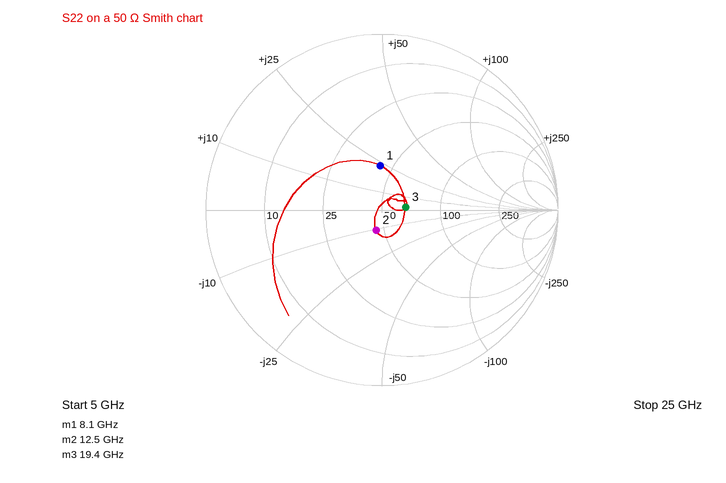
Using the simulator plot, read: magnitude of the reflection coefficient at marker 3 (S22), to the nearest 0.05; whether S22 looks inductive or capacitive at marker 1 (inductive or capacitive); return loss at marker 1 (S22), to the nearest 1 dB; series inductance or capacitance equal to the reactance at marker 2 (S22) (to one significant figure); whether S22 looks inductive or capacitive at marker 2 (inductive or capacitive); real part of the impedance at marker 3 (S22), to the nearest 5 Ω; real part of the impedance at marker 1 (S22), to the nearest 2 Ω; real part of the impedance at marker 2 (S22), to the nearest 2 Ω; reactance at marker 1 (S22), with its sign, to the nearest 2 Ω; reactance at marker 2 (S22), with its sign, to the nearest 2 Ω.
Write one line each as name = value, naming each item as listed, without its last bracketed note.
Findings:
magnitude of the reflection coefficient at marker 3 (S22), to the nearest 0.05 = 0.15
whether S22 looks inductive or capacitive at marker 1 = inductive
return loss at marker 1 (S22), to the nearest 1 dB = 12 dB
series inductance or capacitance equal to the reactance at marker 2 (S22) = 1 pF
whether S22 looks inductive or capacitive at marker 2 = capacitive
real part of the impedance at marker 3 (S22), to the nearest 5 Ω = 65 Ω
real part of the impedance at marker 1 (S22), to the nearest 2 Ω = 44 Ω
real part of the impedance at marker 2 (S22), to the nearest 2 Ω = 46 Ω
reactance at marker 1 (S22), with its sign, to the nearest 2 Ω = +24 Ω
reactance at marker 2 (S22), with its sign, to the nearest 2 Ω = -10 Ω
